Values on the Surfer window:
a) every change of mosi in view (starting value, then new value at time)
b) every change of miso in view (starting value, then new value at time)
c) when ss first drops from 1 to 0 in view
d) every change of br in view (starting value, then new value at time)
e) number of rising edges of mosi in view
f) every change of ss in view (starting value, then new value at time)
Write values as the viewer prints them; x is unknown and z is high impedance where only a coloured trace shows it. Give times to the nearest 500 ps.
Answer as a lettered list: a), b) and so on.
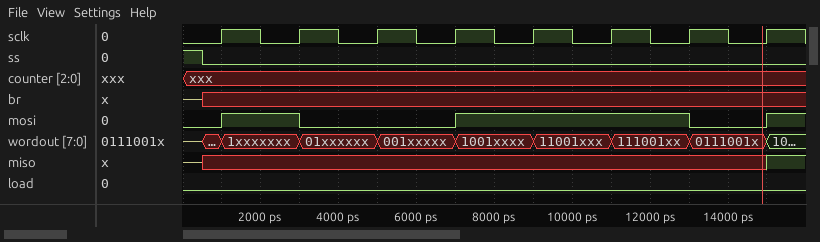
a) 0, 1 at 1000 ps, 0 at 3000 ps, 1 at 7000 ps, 0 at 13000 ps, 1 at 15000 ps
b) z, x at 500 ps, 1 at 15000 ps
c) 500 ps
d) z, x at 500 ps
e) 3
f) 1, 0 at 500 ps
